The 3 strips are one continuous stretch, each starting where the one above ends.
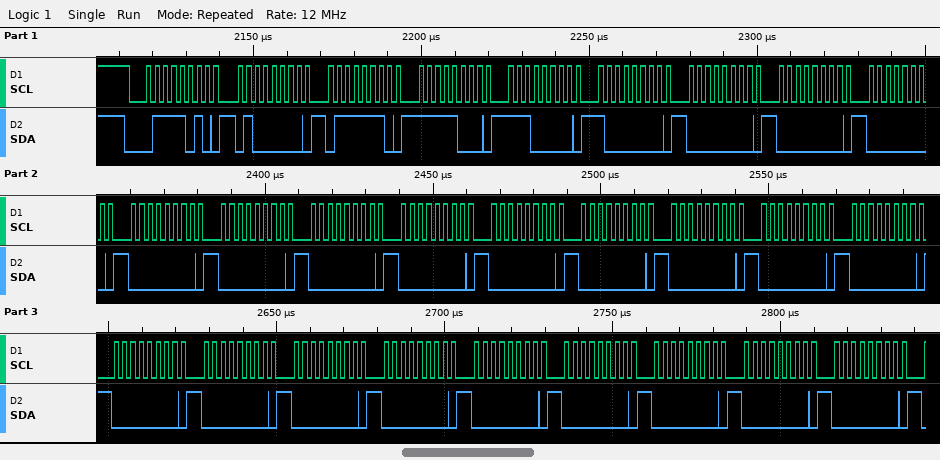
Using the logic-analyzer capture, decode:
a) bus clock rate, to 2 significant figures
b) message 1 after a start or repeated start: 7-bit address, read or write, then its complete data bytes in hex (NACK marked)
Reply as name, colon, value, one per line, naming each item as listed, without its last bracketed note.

bus clock rate, to 2 significant figures: 400 kHz
message 1 after a start or repeated start: 7-bit address, read or write, then its complete data bytes in hex: 0x3D write: 40 7E F8 E0 80 00 00 00 00 00 00 00 00 00 00 00 00 00 00 00 00 00 00 00 00 00
